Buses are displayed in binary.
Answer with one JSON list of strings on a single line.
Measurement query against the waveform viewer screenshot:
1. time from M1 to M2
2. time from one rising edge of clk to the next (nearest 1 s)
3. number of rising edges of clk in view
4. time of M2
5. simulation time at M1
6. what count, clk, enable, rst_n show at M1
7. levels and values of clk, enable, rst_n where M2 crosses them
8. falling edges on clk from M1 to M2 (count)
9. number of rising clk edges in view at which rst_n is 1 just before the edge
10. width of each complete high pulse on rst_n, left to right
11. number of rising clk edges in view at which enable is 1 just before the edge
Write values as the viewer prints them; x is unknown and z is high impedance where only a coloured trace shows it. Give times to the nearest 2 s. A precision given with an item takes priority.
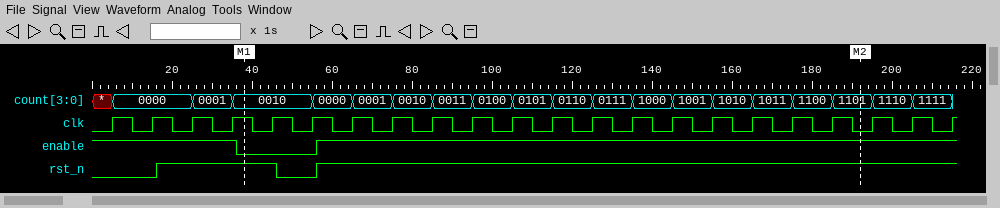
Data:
["154 s", "10 s", "22", "192 s", "38 s", "count=0010, clk=1, enable=0, rst_n=1", "clk=0, enable=1, rst_n=1", "16", "19", "30 s", "20"]
